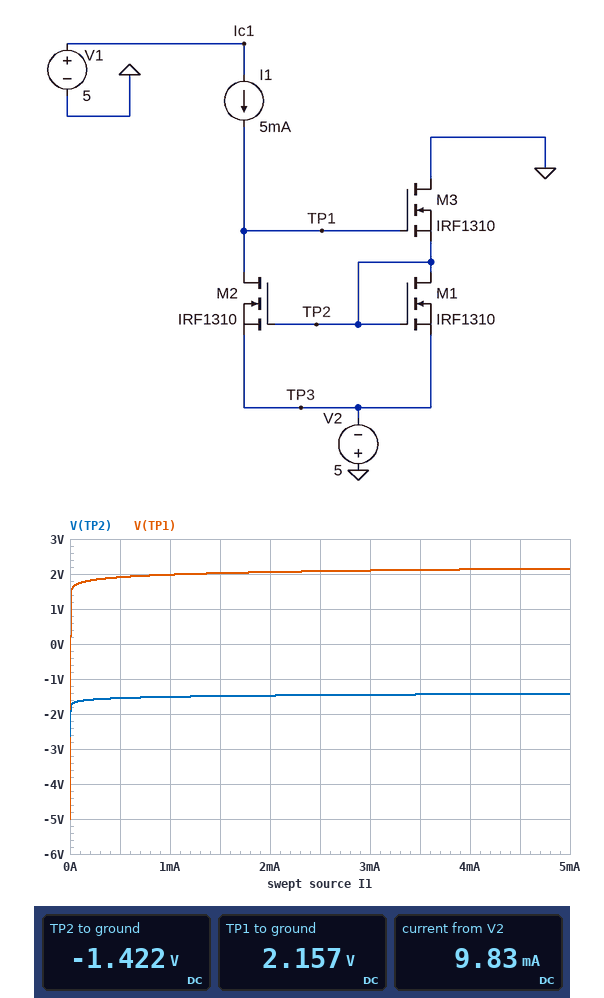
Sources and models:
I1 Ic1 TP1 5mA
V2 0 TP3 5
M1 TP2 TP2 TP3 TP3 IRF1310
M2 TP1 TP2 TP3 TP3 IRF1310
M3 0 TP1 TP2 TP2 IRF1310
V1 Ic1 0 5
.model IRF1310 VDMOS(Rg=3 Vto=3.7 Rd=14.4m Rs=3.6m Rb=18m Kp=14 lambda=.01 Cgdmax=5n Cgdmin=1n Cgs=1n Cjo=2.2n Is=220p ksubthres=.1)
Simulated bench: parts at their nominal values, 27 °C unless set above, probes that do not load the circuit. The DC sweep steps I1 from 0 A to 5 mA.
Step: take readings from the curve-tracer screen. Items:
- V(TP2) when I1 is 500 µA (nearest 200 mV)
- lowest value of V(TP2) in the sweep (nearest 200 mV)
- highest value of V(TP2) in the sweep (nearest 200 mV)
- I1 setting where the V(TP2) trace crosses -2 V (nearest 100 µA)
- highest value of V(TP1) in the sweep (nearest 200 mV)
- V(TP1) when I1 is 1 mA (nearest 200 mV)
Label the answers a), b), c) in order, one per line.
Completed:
a) -1.6 V
b) -2.6 V
c) -1.4 V
d) 0 A
e) 2.2 V
f) 2.0 V
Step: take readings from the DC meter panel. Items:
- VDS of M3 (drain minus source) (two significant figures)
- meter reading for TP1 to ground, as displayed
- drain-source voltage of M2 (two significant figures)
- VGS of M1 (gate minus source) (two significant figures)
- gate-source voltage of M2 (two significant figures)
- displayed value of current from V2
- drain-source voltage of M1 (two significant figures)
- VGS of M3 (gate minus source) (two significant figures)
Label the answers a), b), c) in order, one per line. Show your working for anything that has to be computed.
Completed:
a) 0 V - (-1.422 V) = 1.4 V
b) 2.157 V
c) 2.157 V - (-5 V) = 7.2 V
d) -1.422 V - (-5 V) = 3.6 V
e) -1.422 V - (-5 V) = 3.6 V
f) 9.83 mA
g) -1.422 V - (-5 V) = 3.6 V
h) 2.157 V - (-1.422 V) = 3.6 V
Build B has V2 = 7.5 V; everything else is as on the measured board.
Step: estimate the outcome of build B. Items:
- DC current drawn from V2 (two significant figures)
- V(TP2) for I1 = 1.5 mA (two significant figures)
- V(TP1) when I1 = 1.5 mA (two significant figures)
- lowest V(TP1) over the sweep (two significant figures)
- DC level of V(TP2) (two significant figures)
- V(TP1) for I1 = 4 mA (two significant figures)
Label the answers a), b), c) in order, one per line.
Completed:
a) 9.8 mA
b) -4.0 V
c) -480 mV
d) -7.5 V
e) -3.9 V
f) -370 mV
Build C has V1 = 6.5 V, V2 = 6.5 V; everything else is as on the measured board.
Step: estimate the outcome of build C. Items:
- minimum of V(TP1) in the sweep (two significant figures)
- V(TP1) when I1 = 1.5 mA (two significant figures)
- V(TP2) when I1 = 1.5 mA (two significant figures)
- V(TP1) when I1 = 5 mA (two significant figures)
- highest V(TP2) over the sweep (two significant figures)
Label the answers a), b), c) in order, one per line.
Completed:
a) -6.5 V
b) 520 mV
c) -3.0 V
d) 660 mV
e) -2.9 V
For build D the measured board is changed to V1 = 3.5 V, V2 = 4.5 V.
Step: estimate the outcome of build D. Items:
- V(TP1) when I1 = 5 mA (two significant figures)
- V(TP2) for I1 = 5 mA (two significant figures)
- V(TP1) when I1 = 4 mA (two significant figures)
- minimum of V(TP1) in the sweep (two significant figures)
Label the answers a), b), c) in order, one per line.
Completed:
a) 2.7 V
b) -920 mV
c) 2.6 V
d) -4.5 V
